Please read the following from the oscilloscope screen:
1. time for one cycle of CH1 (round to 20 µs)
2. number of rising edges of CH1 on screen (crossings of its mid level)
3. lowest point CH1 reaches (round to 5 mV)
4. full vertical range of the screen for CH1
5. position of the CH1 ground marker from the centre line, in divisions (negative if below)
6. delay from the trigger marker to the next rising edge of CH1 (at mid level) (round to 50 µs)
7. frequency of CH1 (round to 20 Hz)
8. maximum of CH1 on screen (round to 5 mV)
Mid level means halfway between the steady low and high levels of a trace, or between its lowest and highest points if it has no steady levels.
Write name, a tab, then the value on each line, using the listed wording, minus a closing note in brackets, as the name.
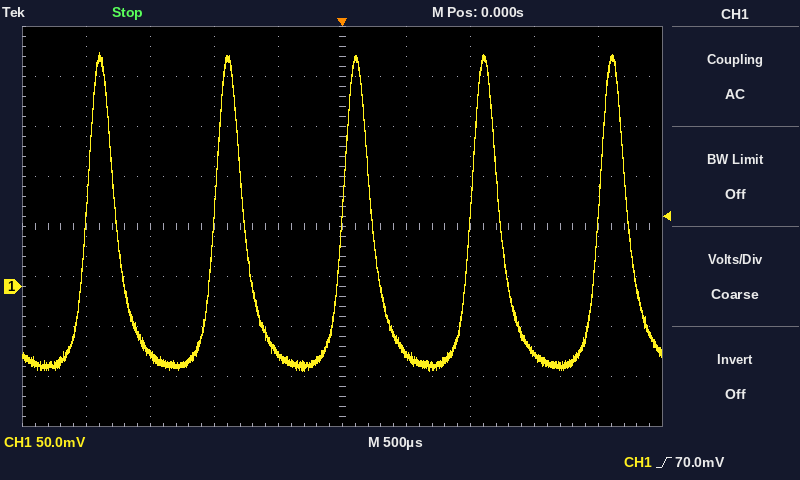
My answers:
time for one cycle of CH1	1.00 ms
number of rising edges of CH1 on screen	5
lowest point CH1 reaches	-85 mV
full vertical range of the screen for CH1	400 mV
position of the CH1 ground marker from the centre line, in divisions	-1.2 div
delay from the trigger marker to the next rising edge of CH1 (at mid level)	1.00 ms
frequency of CH1	1.00 kHz
maximum of CH1 on screen	235 mV
